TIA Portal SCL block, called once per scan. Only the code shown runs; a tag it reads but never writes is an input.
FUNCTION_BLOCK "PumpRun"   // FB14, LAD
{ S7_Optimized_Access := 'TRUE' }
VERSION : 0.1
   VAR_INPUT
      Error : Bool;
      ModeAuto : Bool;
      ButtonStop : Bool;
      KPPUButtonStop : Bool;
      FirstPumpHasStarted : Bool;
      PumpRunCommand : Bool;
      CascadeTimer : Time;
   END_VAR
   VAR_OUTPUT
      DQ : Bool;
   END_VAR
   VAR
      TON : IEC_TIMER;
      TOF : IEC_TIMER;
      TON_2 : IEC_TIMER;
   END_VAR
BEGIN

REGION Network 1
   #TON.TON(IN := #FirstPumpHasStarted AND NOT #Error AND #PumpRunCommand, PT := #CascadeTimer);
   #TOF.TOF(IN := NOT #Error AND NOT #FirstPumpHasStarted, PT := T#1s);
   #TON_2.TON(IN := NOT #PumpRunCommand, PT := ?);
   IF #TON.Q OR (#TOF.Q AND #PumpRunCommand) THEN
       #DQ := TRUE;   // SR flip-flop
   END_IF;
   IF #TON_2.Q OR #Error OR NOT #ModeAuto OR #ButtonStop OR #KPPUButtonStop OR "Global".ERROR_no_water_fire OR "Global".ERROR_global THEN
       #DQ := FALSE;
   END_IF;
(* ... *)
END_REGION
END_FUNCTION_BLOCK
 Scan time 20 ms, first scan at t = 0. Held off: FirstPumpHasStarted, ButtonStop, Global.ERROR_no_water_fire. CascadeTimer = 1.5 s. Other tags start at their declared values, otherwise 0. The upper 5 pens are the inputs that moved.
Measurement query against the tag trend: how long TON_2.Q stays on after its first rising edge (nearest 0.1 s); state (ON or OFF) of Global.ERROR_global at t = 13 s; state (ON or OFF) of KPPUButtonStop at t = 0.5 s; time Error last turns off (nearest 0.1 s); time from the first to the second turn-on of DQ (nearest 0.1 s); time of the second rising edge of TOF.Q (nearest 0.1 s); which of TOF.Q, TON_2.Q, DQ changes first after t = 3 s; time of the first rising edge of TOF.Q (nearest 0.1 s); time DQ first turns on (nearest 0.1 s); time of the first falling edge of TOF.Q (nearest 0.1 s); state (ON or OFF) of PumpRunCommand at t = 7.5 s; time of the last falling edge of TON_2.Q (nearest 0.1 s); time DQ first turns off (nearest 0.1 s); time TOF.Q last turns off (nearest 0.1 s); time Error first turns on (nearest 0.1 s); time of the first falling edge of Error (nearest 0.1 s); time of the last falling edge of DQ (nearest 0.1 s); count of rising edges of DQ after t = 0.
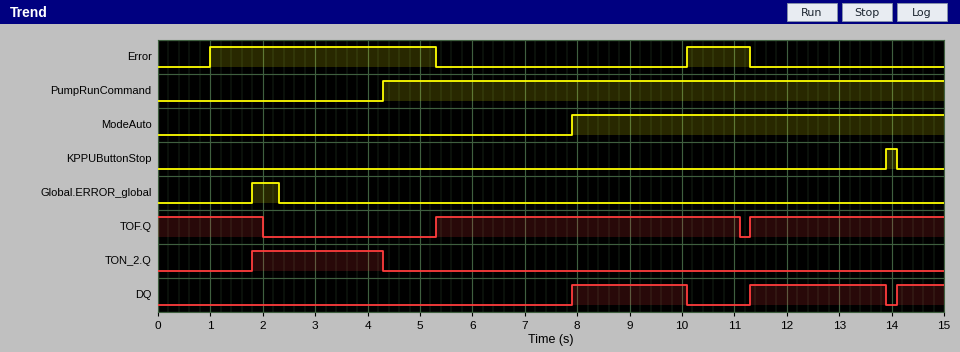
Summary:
2.5 s
OFF
OFF
11.3 s
3.4 s
11.3 s
TON_2.Q
5.3 s
7.9 s
2.0 s
ON
4.3 s
10.1 s
11.1 s
1.0 s
5.3 s
13.9 s
3
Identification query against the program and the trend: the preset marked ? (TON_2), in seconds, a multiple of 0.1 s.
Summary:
1.8 s
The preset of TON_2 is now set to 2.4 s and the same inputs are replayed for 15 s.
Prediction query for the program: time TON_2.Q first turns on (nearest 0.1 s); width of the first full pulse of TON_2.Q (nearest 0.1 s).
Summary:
2.4 s
1.9 s
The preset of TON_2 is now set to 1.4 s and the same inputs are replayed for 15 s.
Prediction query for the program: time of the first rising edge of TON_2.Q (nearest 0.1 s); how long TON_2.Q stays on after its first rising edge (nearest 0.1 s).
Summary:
1.4 s
2.9 s
